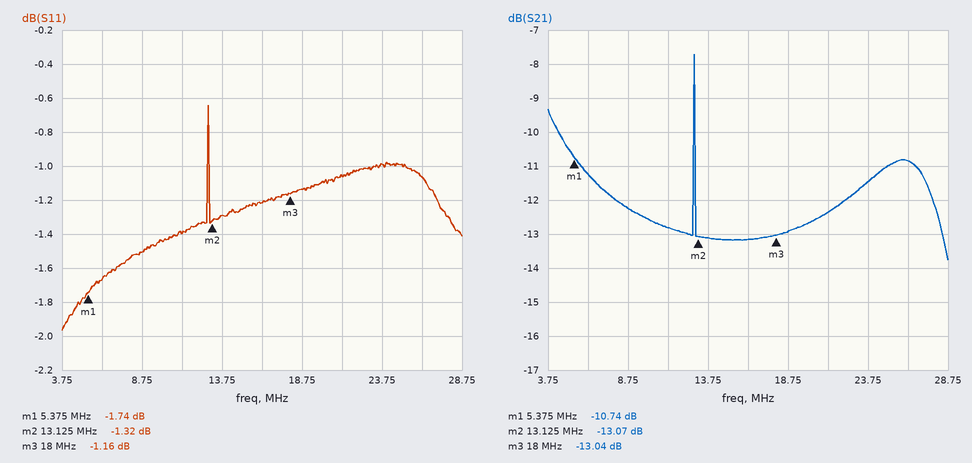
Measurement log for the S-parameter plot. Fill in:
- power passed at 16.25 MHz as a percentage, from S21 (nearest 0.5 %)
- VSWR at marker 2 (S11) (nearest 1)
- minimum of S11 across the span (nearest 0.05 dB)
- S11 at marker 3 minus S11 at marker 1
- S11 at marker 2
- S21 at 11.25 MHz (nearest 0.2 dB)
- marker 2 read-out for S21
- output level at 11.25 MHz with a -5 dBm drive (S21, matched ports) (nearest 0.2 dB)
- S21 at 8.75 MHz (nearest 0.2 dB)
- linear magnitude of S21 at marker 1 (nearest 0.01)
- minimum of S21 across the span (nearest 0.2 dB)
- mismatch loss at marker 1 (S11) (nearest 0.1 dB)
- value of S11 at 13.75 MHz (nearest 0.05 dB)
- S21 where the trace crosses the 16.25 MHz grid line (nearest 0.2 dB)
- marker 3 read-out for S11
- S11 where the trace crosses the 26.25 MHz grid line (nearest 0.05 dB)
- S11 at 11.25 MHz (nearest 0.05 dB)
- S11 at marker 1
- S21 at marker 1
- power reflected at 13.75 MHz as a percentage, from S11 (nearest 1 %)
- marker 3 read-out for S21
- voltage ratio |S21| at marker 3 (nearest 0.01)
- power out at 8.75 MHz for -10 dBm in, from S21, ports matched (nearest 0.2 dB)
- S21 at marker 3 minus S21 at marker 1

5.0 %
13
-1.95 dB
0.58 dB
-1.32 dB
-12.8 dB
-13.07 dB
-17.8 dBm
-12.2 dB
0.29
-13.8 dB
4.8 dB
-1.30 dB
-13.2 dB
-1.16 dB
-1.05 dB
-1.40 dB
-1.74 dB
-10.74 dB
74 %
-13.04 dB
0.22
-22.2 dBm
-2.30 dB
